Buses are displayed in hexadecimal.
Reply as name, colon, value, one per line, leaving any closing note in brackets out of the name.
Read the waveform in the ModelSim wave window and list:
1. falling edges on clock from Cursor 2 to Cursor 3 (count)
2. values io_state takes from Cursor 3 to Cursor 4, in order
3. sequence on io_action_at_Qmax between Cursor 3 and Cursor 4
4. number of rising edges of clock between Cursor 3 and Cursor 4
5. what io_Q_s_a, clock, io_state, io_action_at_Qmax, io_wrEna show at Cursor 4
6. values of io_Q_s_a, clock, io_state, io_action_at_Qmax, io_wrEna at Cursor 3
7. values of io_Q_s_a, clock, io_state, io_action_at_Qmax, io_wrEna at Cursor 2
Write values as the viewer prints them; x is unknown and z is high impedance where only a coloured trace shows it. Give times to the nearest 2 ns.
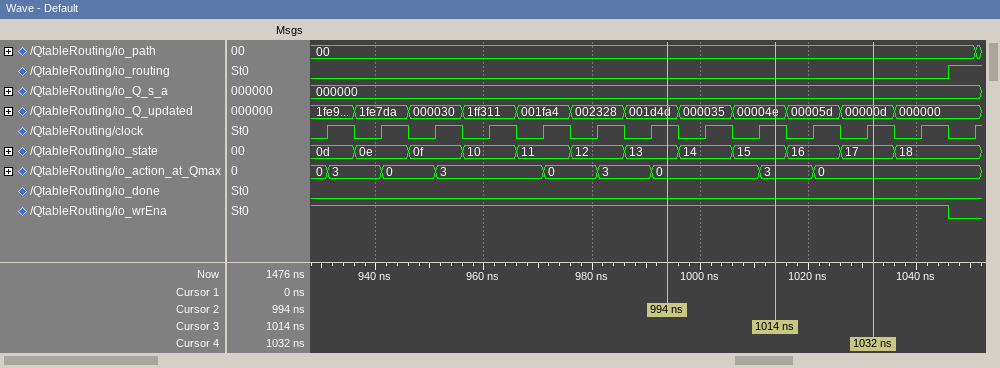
falling edges on clock from Cursor 2 to Cursor 3: 2
values io_state takes from Cursor 3 to Cursor 4, in order: 15, 16, 17
sequence on io_action_at_Qmax between Cursor 3 and Cursor 4: 3, 0
number of rising edges of clock between Cursor 3 and Cursor 4: 2
what io_Q_s_a, clock, io_state, io_action_at_Qmax, io_wrEna show at Cursor 4: io_Q_s_a=000000, clock=1, io_state=17, io_action_at_Qmax=0, io_wrEna=1
values of io_Q_s_a, clock, io_state, io_action_at_Qmax, io_wrEna at Cursor 3: io_Q_s_a=000000, clock=1, io_state=15, io_action_at_Qmax=3, io_wrEna=1
values of io_Q_s_a, clock, io_state, io_action_at_Qmax, io_wrEna at Cursor 2: io_Q_s_a=000000, clock=1, io_state=13, io_action_at_Qmax=0, io_wrEna=1
